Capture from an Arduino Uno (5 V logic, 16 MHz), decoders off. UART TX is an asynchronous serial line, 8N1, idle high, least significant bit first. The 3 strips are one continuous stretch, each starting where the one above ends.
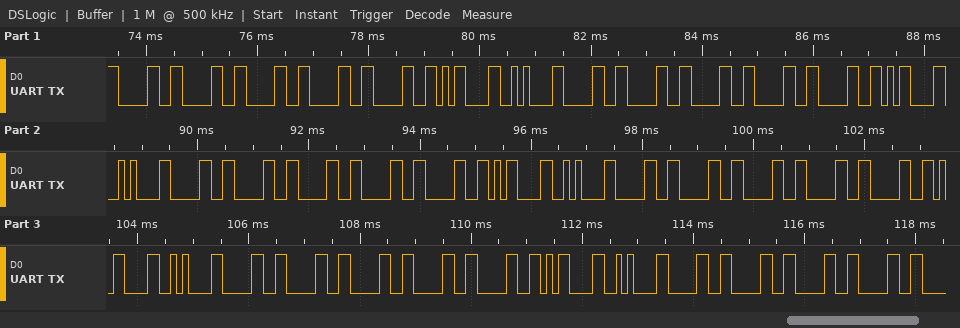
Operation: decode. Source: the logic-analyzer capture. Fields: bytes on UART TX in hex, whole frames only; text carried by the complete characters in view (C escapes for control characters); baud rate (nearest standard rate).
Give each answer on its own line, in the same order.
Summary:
30 30 30 30 30 0D 0A 30 30 30 30 30 0D 0A 30 30 30 30 30 0D 0A 30 30 30 30 30 0D 0A 30 30 30 30 30 0D 0A 30 30 30 30
"00000\r\n00000\r\n00000\r\n00000\r\n00000\r\n0000"
9600 baud
